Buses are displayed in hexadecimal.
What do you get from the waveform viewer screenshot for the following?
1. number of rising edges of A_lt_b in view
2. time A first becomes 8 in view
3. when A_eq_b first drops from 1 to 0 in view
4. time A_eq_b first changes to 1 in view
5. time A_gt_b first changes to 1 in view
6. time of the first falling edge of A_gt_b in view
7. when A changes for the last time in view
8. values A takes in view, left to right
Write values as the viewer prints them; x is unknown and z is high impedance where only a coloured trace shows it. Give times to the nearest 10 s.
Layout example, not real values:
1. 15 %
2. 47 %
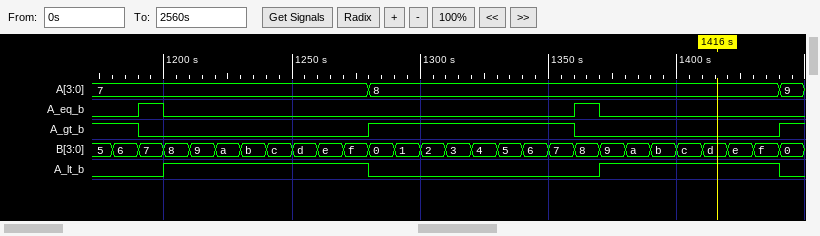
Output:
1. 2
2. 1280 s
3. 1200 s
4. 1190 s
5. 1280 s
6. 1190 s
7. 1440 s
8. 7, 8, 9
